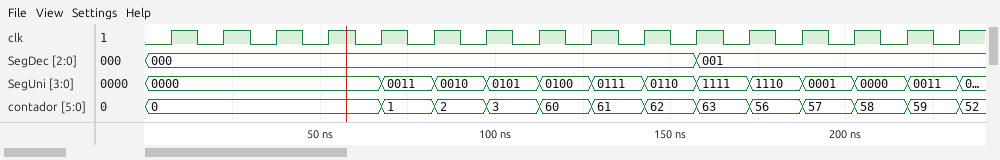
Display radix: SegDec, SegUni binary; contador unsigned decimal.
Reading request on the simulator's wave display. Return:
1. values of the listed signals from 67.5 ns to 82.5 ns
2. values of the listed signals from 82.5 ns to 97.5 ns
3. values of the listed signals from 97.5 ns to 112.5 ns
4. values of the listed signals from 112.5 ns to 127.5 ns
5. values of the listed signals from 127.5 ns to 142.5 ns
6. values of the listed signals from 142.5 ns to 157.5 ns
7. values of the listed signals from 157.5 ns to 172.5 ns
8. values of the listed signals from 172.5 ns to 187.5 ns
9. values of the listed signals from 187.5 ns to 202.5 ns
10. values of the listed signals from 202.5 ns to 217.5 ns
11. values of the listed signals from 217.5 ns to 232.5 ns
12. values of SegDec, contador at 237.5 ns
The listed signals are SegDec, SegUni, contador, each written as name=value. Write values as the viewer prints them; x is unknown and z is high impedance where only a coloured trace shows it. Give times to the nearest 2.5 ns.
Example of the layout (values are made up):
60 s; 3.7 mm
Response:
SegDec=000, SegUni=0011, contador=1; SegDec=000, SegUni=0010, contador=2; SegDec=000, SegUni=0101, contador=3; SegDec=000, SegUni=0100, contador=60; SegDec=000, SegUni=0111, contador=61; SegDec=000, SegUni=0110, contador=62; SegDec=001, SegUni=1111, contador=63; SegDec=001, SegUni=1110, contador=56; SegDec=001, SegUni=0001, contador=57; SegDec=001, SegUni=0000, contador=58; SegDec=001, SegUni=0011, contador=59; SegDec=001, contador=52
